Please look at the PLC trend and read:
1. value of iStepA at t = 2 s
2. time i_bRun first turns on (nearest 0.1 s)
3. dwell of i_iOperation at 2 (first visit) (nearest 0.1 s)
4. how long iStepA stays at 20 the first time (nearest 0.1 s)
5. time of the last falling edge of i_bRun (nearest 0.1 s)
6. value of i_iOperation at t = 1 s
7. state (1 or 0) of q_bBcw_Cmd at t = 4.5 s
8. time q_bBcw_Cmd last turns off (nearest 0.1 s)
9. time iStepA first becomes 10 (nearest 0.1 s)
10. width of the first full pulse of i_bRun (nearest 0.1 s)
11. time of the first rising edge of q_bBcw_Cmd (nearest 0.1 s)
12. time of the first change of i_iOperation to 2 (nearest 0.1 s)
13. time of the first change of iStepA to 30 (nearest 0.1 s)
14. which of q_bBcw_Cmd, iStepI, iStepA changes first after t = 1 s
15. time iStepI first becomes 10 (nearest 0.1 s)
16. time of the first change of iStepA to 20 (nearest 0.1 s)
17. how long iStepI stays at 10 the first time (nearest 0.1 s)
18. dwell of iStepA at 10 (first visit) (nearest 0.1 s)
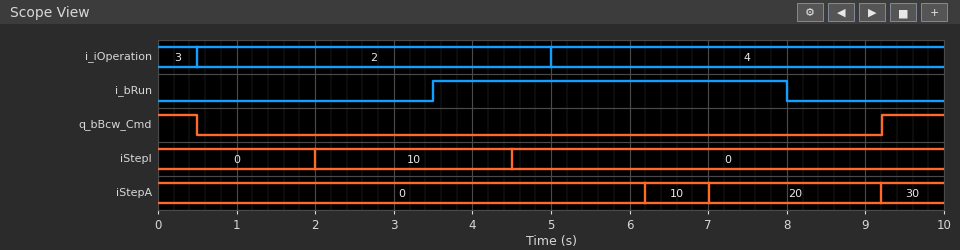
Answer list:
0
3.5 s
4.5 s
2.2 s
8.0 s
2
0
0.5 s
6.2 s
4.5 s
9.2 s
0.5 s
9.2 s
iStepI
2.0 s
7.0 s
2.5 s
0.8 s
